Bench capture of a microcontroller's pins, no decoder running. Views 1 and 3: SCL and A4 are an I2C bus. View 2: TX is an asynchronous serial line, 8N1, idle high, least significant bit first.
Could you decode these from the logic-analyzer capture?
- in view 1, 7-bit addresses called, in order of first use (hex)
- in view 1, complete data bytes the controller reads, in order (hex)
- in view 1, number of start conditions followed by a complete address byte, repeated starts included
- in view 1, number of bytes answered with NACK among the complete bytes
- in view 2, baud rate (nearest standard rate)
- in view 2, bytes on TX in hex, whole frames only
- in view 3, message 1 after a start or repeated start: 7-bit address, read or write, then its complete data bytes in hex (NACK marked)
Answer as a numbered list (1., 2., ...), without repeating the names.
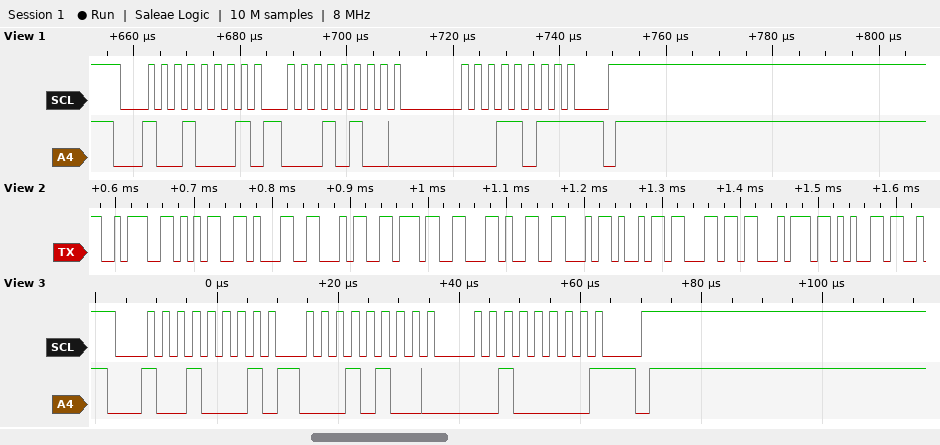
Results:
1. 0x48
2. 14 1B
3. 1
4. 1
5. 115200 baud
6. 3A 35 31 34 37 2C 46 69 6C 74 65
7. 0x48 read: 14 20 NACK
